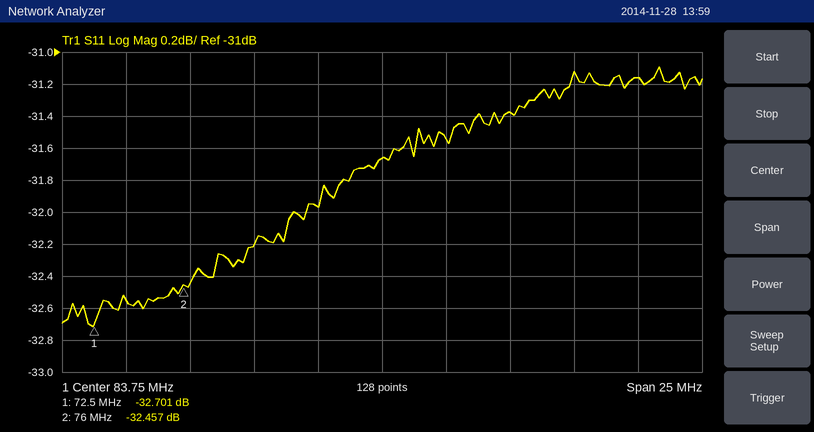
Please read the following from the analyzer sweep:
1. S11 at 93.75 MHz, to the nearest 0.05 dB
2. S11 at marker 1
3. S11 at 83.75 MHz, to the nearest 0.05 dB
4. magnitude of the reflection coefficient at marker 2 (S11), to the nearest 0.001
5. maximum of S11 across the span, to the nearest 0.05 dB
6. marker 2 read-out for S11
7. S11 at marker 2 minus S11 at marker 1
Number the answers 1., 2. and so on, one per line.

1. -31.15 dB
2. -32.701 dB
3. -31.65 dB
4. 0.024
5. -31.10 dB
6. -32.457 dB
7. 0.244 dB
